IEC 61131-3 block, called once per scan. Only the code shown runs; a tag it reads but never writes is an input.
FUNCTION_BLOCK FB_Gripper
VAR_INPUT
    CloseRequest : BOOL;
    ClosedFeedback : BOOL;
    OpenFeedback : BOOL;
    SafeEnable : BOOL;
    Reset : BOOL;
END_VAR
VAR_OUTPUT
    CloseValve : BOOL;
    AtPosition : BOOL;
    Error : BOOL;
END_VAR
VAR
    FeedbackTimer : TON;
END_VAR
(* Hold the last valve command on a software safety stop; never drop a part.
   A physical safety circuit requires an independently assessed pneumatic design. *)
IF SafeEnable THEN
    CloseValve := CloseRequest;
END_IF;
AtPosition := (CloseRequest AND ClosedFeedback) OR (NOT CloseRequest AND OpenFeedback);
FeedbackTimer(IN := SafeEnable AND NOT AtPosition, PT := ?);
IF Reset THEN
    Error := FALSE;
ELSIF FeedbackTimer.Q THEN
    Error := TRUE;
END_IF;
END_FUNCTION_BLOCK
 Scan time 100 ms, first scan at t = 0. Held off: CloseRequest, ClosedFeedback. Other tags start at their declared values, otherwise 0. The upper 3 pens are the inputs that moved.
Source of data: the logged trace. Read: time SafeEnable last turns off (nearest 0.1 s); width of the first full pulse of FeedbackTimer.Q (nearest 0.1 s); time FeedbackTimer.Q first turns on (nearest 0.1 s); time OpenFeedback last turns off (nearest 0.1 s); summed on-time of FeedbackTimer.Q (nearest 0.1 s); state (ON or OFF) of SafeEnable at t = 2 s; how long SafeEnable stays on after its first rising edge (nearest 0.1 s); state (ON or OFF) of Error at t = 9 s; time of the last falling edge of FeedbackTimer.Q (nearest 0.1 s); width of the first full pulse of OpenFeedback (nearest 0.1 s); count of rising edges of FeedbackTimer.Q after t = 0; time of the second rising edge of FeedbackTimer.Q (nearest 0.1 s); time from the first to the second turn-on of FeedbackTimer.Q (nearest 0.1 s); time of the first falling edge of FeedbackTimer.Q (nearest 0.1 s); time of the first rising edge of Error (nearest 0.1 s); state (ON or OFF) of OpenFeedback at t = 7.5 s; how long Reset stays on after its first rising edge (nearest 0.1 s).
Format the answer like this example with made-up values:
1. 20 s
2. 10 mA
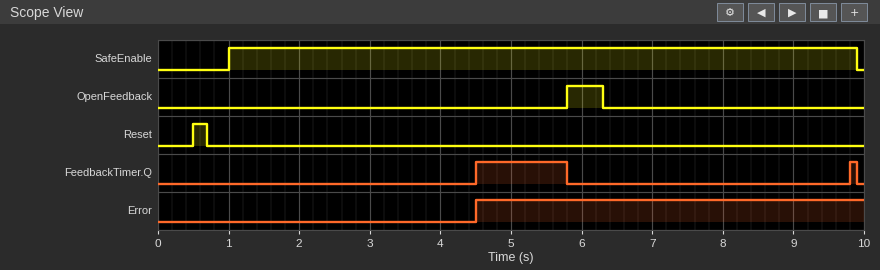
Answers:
1. 9.9 s
2. 1.3 s
3. 4.5 s
4. 6.3 s
5. 1.4 s
6. ON
7. 8.9 s
8. ON
9. 9.9 s
10. 0.5 s
11. 2
12. 9.8 s
13. 5.3 s
14. 5.8 s
15. 4.5 s
16. OFF
17. 0.2 s
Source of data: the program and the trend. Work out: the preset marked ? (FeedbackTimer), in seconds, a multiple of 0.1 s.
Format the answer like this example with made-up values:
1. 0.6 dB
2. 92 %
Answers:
1. 3.5 s
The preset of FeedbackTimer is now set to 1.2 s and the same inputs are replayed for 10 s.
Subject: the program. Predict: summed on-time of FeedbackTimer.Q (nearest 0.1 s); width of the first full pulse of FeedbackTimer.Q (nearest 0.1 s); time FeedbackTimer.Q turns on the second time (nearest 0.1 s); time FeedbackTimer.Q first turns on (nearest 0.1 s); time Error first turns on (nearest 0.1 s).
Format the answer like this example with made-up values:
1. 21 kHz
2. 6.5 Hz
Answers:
1. 6.0 s
2. 3.6 s
3. 7.5 s
4. 2.2 s
5. 2.2 s
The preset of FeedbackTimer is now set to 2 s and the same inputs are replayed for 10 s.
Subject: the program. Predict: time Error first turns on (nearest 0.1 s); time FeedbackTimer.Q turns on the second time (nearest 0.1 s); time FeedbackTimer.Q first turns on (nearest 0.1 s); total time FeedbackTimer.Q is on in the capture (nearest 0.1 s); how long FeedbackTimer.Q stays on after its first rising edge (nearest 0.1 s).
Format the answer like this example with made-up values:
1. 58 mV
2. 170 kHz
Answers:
1. 3.0 s
2. 8.3 s
3. 3.0 s
4. 4.4 s
5. 2.8 s
